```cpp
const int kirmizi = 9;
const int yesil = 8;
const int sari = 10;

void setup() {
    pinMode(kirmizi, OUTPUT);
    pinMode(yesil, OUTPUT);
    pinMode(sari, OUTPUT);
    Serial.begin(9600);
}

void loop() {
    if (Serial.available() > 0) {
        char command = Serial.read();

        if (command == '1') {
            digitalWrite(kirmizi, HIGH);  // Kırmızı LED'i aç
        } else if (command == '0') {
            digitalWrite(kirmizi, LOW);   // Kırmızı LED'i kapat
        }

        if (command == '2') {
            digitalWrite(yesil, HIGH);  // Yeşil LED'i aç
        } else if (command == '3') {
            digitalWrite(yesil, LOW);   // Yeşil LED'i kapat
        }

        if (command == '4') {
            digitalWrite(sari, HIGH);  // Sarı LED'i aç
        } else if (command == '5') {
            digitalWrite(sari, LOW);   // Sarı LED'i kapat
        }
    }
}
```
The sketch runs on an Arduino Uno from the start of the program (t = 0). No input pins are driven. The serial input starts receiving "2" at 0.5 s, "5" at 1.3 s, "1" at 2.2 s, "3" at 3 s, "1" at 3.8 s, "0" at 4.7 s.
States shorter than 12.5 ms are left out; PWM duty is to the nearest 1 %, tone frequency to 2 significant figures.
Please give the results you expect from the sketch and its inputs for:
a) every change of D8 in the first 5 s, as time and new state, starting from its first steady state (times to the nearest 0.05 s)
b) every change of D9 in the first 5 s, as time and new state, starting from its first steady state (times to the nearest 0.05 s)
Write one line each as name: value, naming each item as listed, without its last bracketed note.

every change of D8 in the first 5 s, as time and new state, starting from its first steady state: 0 s low; 0.5 s high; 3 s low
every change of D9 in the first 5 s, as time and new state, starting from its first steady state: 0 s low; 2.2 s high; 4.7 s low
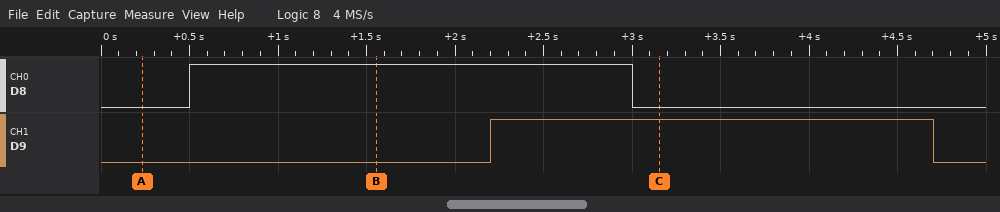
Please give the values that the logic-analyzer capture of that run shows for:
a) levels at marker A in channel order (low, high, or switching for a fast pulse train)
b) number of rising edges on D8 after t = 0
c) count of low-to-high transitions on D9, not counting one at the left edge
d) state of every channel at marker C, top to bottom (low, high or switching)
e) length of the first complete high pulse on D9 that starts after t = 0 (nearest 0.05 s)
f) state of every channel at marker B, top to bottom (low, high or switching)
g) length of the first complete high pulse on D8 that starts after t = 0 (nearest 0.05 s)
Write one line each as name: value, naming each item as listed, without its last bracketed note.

levels at marker A in channel order: D8 low, D9 low
number of rising edges on D8 after t = 0: 1
count of low-to-high transitions on D9, not counting one at the left edge: 1
state of every channel at marker C, top to bottom: D8 low, D9 high
length of the first complete high pulse on D9 that starts after t = 0: 2.50 s
state of every channel at marker B, top to bottom: D8 high, D9 low
length of the first complete high pulse on D8 that starts after t = 0: 2.50 s
